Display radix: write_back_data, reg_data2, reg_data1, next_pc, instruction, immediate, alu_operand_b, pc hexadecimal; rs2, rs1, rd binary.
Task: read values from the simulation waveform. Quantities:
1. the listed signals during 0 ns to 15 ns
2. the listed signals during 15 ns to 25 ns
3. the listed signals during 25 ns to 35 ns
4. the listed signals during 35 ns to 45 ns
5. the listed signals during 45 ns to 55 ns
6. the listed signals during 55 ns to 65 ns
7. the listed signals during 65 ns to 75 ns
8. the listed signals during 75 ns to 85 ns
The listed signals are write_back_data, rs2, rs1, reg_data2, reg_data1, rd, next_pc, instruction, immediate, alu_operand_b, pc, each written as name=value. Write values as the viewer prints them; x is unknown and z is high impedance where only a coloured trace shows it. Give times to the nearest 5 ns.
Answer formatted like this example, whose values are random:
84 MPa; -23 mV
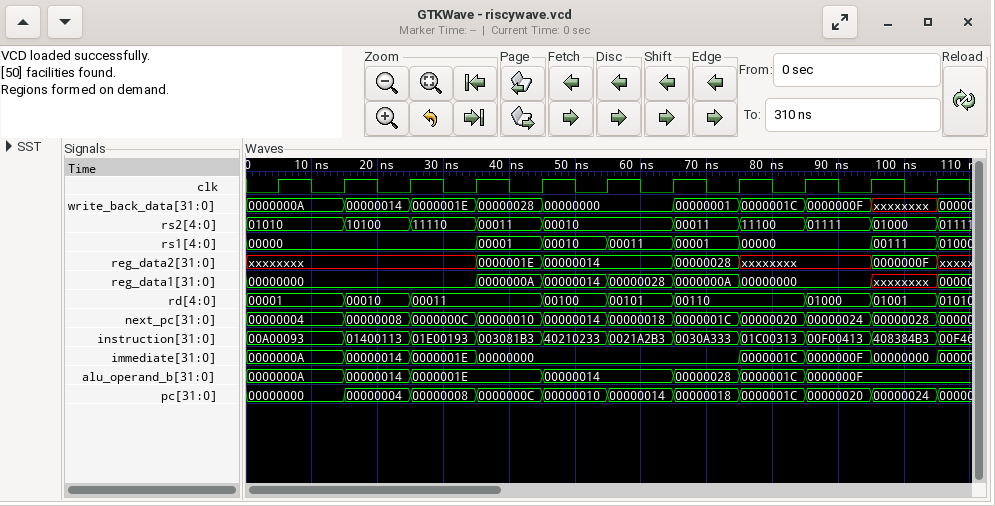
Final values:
write_back_data=0000000A, rs2=01010, rs1=00000, reg_data2=xxxxxxxx, reg_data1=00000000, rd=00001, next_pc=00000004, instruction=00A00093, immediate=0000000A, alu_operand_b=0000000A, pc=00000000; write_back_data=00000014, rs2=10100, rs1=00000, reg_data2=xxxxxxxx, reg_data1=00000000, rd=00010, next_pc=00000008, instruction=01400113, immediate=00000014, alu_operand_b=00000014, pc=00000004; write_back_data=0000001E, rs2=11110, rs1=00000, reg_data2=xxxxxxxx, reg_data1=00000000, rd=00011, next_pc=0000000C, instruction=01E00193, immediate=0000001E, alu_operand_b=0000001E, pc=00000008; write_back_data=00000028, rs2=00011, rs1=00001, reg_data2=0000001E, reg_data1=0000000A, rd=00011, next_pc=00000010, instruction=003081B3, immediate=00000000, alu_operand_b=0000001E, pc=0000000C; write_back_data=00000000, rs2=00010, rs1=00010, reg_data2=00000014, reg_data1=00000014, rd=00100, next_pc=00000014, instruction=40210233, immediate=00000000, alu_operand_b=00000014, pc=00000010; write_back_data=00000000, rs2=00010, rs1=00011, reg_data2=00000014, reg_data1=00000028, rd=00101, next_pc=00000018, instruction=0021A2B3, immediate=00000000, alu_operand_b=00000014, pc=00000014; write_back_data=00000001, rs2=00011, rs1=00001, reg_data2=00000028, reg_data1=0000000A, rd=00110, next_pc=0000001C, instruction=0030A333, immediate=00000000, alu_operand_b=00000028, pc=00000018; write_back_data=0000001C, rs2=11100, rs1=00000, reg_data2=xxxxxxxx, reg_data1=00000000, rd=00110, next_pc=00000020, instruction=01C00313, immediate=0000001C, alu_operand_b=0000001C, pc=0000001C
